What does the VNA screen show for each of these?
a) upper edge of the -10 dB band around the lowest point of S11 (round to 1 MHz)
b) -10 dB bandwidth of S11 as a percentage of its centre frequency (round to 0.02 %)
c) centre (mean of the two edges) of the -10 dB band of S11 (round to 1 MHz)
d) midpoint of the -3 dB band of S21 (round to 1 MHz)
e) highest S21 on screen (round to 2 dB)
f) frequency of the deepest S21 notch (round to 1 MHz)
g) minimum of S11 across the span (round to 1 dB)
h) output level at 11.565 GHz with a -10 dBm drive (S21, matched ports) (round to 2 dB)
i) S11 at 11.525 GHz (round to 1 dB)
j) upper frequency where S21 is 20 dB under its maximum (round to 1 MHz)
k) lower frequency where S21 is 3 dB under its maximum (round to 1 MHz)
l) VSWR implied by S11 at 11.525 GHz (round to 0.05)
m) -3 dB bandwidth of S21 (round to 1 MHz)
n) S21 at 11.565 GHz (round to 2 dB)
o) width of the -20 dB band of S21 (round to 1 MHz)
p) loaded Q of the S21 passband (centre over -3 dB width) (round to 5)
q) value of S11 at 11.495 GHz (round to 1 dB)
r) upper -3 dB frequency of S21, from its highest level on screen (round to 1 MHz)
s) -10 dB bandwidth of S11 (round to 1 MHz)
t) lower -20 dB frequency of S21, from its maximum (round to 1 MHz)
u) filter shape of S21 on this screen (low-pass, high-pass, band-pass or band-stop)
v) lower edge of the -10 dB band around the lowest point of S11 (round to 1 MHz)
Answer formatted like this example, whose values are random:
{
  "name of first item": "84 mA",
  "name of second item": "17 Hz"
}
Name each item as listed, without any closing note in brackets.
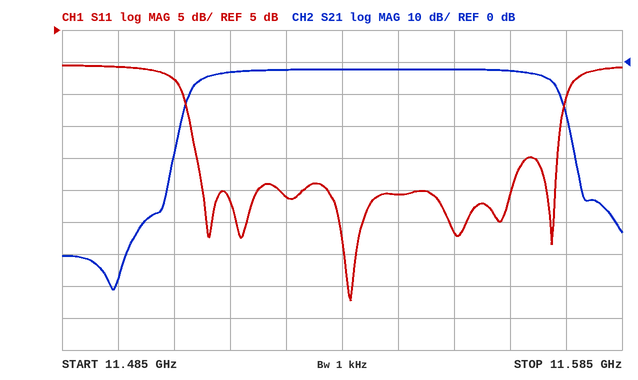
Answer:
{
  "upper edge of the -10 dB band around the lowest point of S11": "11.574 GHz",
  "-10 dB bandwidth of S11 as a percentage of its centre frequency": "0.58 %",
  "centre (mean of the two edges) of the -10 dB band of S11": "11.541 GHz",
  "midpoint of the -3 dB band of S21": "11.541 GHz",
  "highest S21 on screen": "-2 dB",
  "frequency of the deepest S21 notch": "11.494 GHz",
  "minimum of S11 across the span": "-37 dB",
  "output level at 11.565 GHz with a -10 dBm drive (S21, matched ports)": "-12 dBm",
  "S11 at 11.525 GHz": "-21 dB",
  "upper frequency where S21 is 20 dB under its maximum": "11.576 GHz",
  "lower frequency where S21 is 3 dB under its maximum": "11.510 GHz",
  "VSWR implied by S11 at 11.525 GHz": "1.20",
  "-3 dB bandwidth of S21": "62 MHz",
  "S21 at 11.565 GHz": "-2 dB",
  "width of the -20 dB band of S21": "70 MHz",
  "loaded Q of the S21 passband (centre over -3 dB width)": "185",
  "value of S11 at 11.495 GHz": "-1 dB",
  "upper -3 dB frequency of S21, from its highest level on screen": "11.572 GHz",
  "-10 dB bandwidth of S11": "66 MHz",
  "lower -20 dB frequency of S21, from its maximum": "11.506 GHz",
  "filter shape of S21 on this screen": "band-pass",
  "lower edge of the -10 dB band around the lowest point of S11": "11.508 GHz"
}
